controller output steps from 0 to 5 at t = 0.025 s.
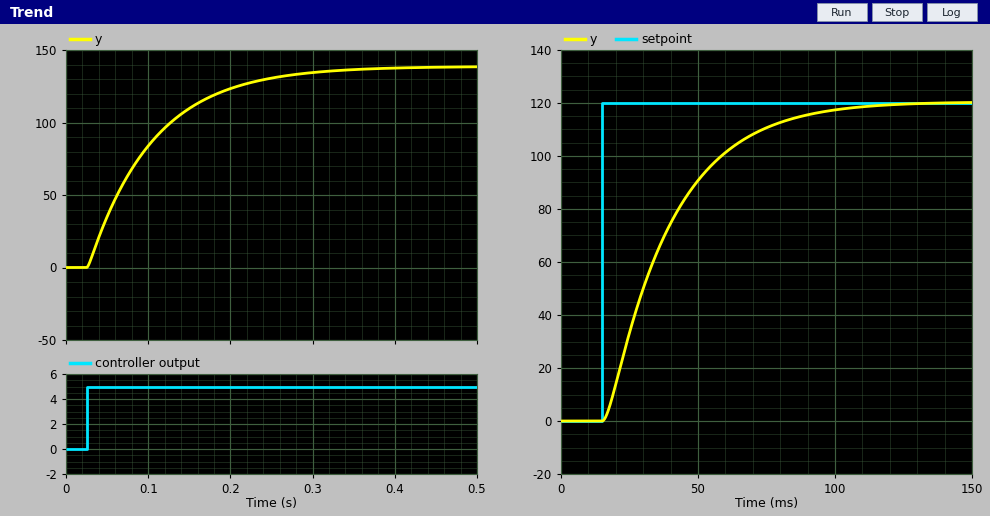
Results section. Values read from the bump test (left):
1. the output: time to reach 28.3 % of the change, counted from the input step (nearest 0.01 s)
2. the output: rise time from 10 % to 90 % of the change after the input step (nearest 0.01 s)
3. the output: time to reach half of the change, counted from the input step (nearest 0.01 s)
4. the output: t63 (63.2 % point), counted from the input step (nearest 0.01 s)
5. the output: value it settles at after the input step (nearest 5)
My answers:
0.03 s
0.17 s
0.06 s
0.08 s
140
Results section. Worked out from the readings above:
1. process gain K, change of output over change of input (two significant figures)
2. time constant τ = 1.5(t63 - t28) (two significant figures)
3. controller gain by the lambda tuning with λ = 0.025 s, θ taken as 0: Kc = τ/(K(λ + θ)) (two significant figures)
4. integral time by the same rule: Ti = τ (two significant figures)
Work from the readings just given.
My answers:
28
0.075 s
0.11
0.075 s
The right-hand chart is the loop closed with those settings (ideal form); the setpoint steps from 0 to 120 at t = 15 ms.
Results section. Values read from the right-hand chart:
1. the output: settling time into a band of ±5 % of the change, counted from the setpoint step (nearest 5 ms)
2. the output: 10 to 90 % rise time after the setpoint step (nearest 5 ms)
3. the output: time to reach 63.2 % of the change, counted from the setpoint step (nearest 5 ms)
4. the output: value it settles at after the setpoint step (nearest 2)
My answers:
70 ms
50 ms
25 ms
120
